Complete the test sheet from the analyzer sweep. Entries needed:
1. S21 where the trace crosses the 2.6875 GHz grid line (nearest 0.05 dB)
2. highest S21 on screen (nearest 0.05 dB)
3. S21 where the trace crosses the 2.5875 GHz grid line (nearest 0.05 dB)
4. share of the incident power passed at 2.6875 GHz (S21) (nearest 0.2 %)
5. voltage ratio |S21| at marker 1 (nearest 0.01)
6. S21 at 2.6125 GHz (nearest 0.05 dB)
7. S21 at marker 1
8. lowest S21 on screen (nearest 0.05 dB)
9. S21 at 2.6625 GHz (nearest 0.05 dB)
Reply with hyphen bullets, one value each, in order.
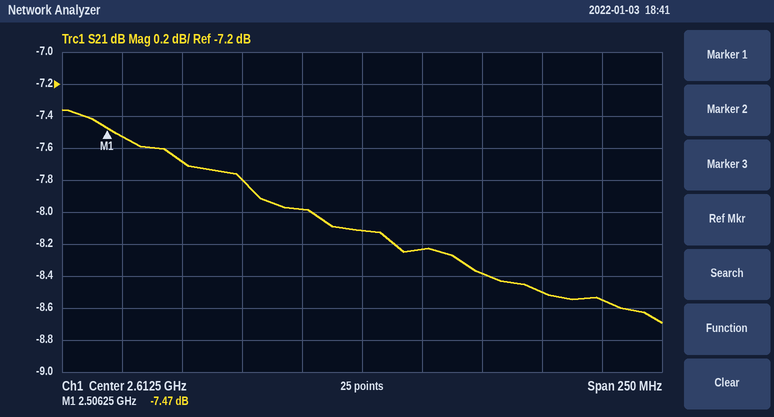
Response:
- -8.50 dB
- -7.35 dB
- -8.00 dB
- 14.2 %
- 0.42
- -8.10 dB
- -7.47 dB
- -8.70 dB
- -8.40 dB
